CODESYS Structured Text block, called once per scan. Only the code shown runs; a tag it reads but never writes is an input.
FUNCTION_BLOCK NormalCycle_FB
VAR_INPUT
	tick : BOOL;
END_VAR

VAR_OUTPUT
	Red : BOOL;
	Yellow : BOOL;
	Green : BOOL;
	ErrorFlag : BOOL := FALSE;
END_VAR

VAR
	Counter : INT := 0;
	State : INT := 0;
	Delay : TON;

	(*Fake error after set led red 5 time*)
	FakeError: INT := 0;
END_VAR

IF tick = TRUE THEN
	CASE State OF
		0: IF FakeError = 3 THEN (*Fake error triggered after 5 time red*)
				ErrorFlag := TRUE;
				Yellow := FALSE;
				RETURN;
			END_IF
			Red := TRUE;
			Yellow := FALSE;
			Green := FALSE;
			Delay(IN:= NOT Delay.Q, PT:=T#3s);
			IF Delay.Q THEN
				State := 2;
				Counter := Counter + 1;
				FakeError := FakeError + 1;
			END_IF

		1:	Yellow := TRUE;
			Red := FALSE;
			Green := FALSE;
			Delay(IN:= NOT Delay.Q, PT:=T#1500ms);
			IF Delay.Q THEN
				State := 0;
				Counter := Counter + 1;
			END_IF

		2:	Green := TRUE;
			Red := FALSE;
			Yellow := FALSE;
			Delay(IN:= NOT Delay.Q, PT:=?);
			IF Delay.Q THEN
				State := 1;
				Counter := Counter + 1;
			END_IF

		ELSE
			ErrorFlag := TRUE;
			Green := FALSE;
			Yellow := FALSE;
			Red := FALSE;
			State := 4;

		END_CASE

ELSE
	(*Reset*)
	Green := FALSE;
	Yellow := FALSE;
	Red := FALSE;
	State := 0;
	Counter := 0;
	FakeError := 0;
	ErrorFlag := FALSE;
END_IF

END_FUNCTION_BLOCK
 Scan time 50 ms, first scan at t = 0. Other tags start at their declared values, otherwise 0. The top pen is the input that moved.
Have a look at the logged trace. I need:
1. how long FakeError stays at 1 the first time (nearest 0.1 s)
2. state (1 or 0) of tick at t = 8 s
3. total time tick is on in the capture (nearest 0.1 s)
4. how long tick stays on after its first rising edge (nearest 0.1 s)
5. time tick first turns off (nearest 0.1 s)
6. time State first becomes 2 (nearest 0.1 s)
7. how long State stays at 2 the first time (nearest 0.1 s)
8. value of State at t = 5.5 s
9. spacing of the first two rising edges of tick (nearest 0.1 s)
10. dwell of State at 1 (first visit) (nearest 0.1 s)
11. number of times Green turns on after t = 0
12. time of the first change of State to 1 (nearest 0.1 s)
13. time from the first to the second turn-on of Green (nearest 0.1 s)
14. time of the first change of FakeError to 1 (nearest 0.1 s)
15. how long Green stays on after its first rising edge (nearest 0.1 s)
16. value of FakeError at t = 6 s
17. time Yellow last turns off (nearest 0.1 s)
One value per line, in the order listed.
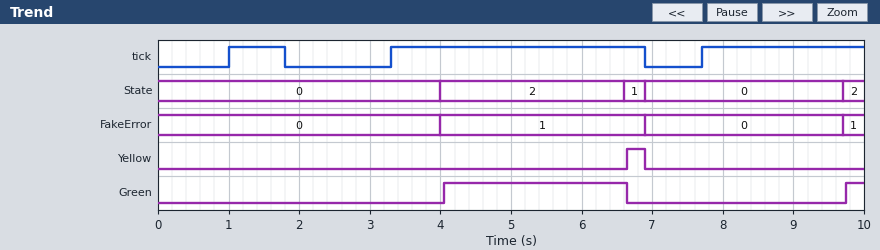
2.9 s
1
6.7 s
0.8 s
1.8 s
4.0 s
2.6 s
2
2.3 s
0.3 s
2
6.6 s
5.7 s
4.0 s
2.6 s
1
6.9 s
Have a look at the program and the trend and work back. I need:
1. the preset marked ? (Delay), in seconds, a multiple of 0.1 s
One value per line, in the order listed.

2.5 s
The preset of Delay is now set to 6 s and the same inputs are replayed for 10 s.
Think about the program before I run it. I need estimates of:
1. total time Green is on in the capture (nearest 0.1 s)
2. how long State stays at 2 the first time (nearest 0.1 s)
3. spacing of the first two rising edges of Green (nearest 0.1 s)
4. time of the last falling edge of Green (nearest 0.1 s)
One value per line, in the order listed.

5.1 s
2.9 s
3.7 s
6.9 s
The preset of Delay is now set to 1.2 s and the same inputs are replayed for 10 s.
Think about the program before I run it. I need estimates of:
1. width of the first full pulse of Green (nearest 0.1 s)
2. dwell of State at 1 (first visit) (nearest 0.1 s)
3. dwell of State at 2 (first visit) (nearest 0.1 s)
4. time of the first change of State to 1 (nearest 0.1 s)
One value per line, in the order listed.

1.3 s
1.6 s
1.3 s
5.3 s
